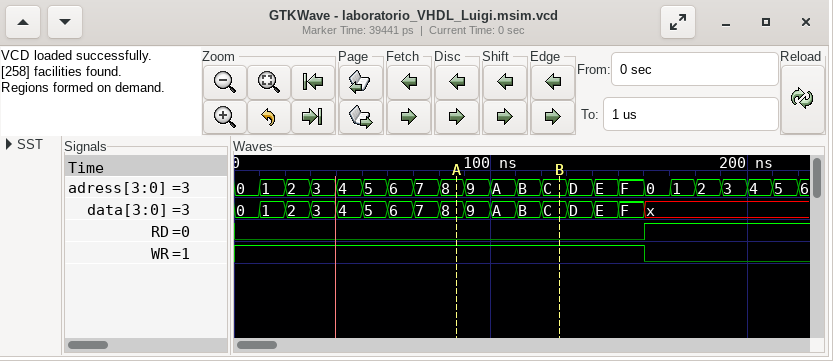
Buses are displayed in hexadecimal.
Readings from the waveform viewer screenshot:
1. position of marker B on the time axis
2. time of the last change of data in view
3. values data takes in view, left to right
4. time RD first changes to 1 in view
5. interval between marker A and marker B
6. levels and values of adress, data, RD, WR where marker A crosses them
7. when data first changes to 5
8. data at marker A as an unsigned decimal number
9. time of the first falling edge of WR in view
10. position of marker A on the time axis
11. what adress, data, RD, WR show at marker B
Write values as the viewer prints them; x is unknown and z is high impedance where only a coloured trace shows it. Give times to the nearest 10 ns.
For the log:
130 ns
160 ns
0, 1, 2, 3, 4, 5, 6, 7, 8, 9, A, B, C, D, E, F, x
160 ns
40 ns
adress=8, data=8, RD=0, WR=1
50 ns
8
160 ns
90 ns
adress=C, data=C, RD=0, WR=1
